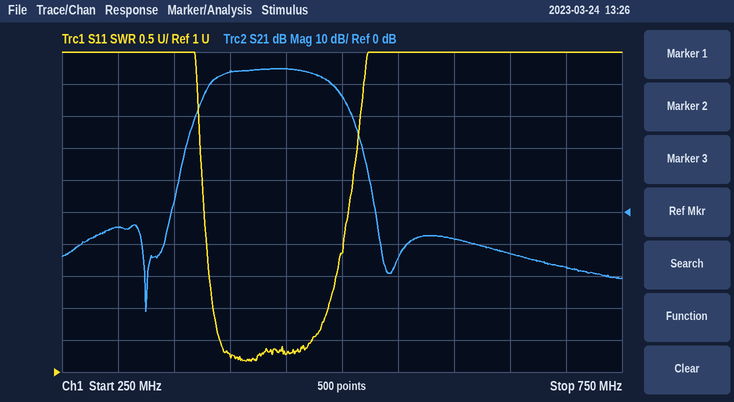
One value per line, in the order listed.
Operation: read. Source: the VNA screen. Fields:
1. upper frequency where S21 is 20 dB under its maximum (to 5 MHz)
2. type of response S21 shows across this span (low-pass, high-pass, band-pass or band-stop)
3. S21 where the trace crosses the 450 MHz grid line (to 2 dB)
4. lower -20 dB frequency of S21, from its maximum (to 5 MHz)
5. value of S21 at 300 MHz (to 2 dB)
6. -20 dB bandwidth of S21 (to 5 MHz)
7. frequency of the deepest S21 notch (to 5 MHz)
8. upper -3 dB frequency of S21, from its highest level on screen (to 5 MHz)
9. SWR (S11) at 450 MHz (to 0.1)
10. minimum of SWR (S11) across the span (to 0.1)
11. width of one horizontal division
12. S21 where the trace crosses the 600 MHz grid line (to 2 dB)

515 MHz
band-pass
44 dB
365 MHz
-4 dB
150 MHz
325 MHz
485 MHz
1.3
1.2
50 MHz
-8 dB
